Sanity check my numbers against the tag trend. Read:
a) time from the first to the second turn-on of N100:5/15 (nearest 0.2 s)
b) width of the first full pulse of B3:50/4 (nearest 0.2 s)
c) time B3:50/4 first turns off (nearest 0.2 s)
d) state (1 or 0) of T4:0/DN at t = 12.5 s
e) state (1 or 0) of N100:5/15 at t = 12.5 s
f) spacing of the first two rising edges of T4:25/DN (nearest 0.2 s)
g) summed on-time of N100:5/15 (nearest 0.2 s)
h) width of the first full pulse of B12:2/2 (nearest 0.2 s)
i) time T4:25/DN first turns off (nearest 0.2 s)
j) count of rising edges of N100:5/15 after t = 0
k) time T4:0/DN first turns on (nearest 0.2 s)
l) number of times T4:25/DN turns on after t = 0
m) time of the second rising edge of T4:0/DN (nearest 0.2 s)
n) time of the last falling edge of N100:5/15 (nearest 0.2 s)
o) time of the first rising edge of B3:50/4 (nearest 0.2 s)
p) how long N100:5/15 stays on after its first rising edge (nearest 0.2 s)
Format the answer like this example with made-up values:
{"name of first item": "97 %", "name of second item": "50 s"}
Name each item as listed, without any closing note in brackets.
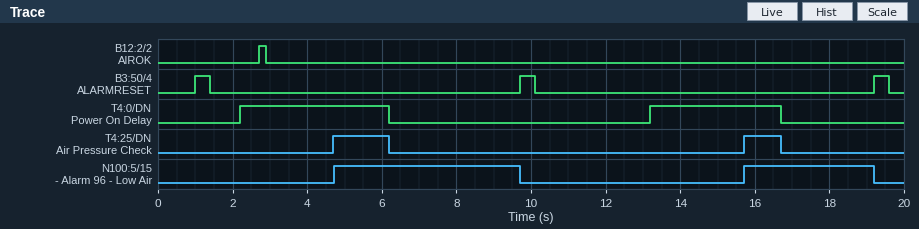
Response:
{"time from the first to the second turn-on of N100:5/15": "11.0 s", "width of the first full pulse of B3:50/4": "0.4 s", "time B3:50/4 first turns off": "1.4 s", "state (1 or 0) of T4:0/DN at t = 12.5 s": "0", "state (1 or 0) of N100:5/15 at t = 12.5 s": "0", "spacing of the first two rising edges of T4:25/DN": "11.0 s", "summed on-time of N100:5/15": "8.4 s", "width of the first full pulse of B12:2/2": "0.2 s", "time T4:25/DN first turns off": "6.2 s", "count of rising edges of N100:5/15 after t = 0": "2", "time T4:0/DN first turns on": "2.2 s", "number of times T4:25/DN turns on after t = 0": "2", "time of the second rising edge of T4:0/DN": "13.2 s", "time of the last falling edge of N100:5/15": "19.2 s", "time of the first rising edge of B3:50/4": "1.0 s", "how long N100:5/15 stays on after its first rising edge": "5.0 s"}
